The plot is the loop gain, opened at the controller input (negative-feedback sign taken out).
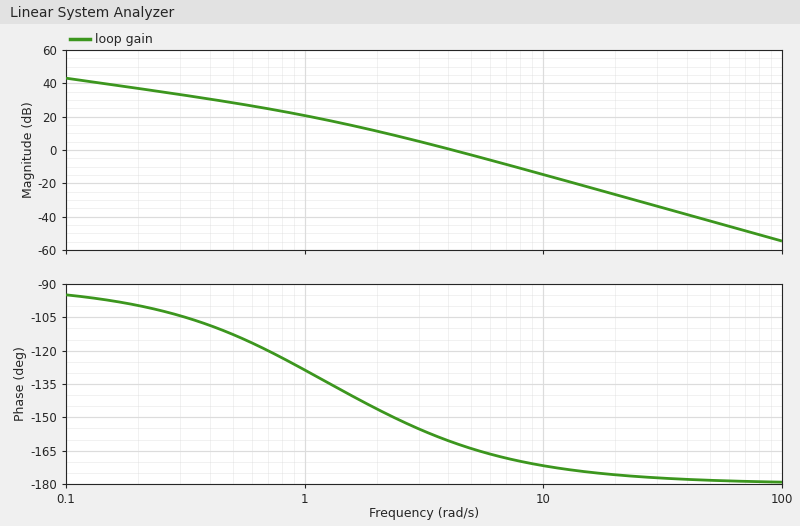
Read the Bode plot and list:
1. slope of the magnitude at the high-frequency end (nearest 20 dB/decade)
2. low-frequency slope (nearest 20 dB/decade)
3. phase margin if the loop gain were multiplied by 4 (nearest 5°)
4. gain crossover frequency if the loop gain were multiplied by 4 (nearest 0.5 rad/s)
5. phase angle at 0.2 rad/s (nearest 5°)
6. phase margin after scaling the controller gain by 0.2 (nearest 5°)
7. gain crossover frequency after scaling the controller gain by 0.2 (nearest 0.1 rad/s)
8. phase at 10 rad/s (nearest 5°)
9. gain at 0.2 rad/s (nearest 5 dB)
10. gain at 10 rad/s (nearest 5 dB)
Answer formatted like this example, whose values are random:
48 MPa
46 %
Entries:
-40 dB/decade
-20 dB/decade
10°
8.5 rad/s
-100°
40°
1.7 rad/s
-170°
35 dB
-15 dB
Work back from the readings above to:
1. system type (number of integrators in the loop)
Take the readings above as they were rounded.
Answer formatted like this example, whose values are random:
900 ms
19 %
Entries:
1
